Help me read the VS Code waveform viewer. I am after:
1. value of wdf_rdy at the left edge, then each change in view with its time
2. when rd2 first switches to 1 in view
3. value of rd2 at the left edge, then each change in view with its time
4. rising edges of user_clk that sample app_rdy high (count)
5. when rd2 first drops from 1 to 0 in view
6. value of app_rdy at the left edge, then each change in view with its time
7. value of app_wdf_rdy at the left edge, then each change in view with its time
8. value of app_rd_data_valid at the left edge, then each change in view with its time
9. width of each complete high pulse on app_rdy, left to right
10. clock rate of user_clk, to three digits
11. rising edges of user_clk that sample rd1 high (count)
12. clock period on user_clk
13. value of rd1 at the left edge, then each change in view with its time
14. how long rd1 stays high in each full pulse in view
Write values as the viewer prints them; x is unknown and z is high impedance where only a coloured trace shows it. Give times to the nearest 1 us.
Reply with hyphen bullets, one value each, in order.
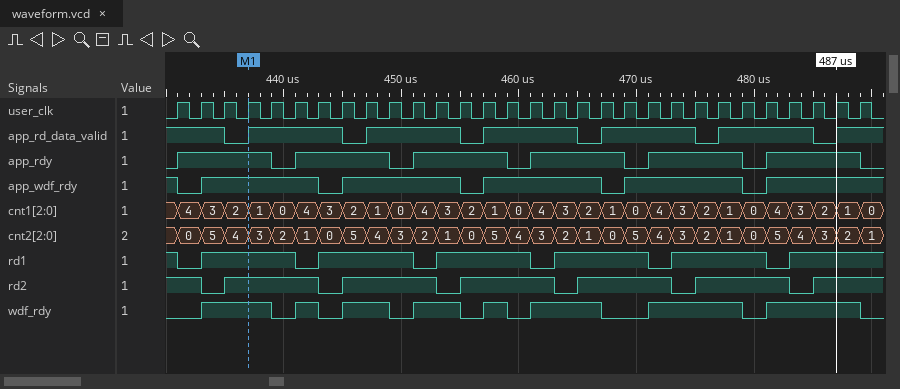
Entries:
- 0, 1 at 433 us, 0 at 439 us, 1 at 441 us, 0 at 443 us, 1 at 445 us, 0 at 449 us, 1 at 451 us, 0 at 455 us, 1 at 457 us, 0 at 459 us, 1 at 461 us, 0 at 467 us, 1 at 471 us, 0 at 479 us, 1 at 481 us, 0 at 489 us
- 435 us
- 1, 0 at 433 us, 1 at 435 us, 0 at 443 us, 1 at 445 us, 0 at 453 us, 1 at 455 us, 0 at 463 us, 1 at 465 us, 0 at 473 us, 1 at 475 us, 0 at 483 us, 1 at 485 us
- 24
- 433 us
- 0, 1 at 431 us, 0 at 439 us, 1 at 441 us, 0 at 449 us, 1 at 451 us, 0 at 459 us, 1 at 461 us, 0 at 469 us, 1 at 471 us, 0 at 479 us, 1 at 481 us, 0 at 489 us
- 1, 0 at 431 us, 1 at 433 us, 0 at 443 us, 1 at 445 us, 0 at 455 us, 1 at 457 us, 0 at 467 us, 1 at 469 us, 0 at 479 us, 1 at 481 us
- 1, 0 at 435 us, 1 at 437 us, 0 at 445 us, 1 at 447 us, 0 at 455 us, 1 at 457 us, 0 at 465 us, 1 at 467 us, 0 at 475 us, 1 at 477 us, 0 at 485 us, 1 at 487 us
- 8 us, 8 us, 8 us, 8 us, 8 us, 8 us
- 500 kHz
- 24
- 2 us
- 1, 0 at 431 us, 1 at 433 us, 0 at 441 us, 1 at 443 us, 0 at 451 us, 1 at 453 us, 0 at 461 us, 1 at 463 us, 0 at 471 us, 1 at 473 us, 0 at 481 us, 1 at 483 us
- 8 us, 8 us, 8 us, 8 us, 8 us
